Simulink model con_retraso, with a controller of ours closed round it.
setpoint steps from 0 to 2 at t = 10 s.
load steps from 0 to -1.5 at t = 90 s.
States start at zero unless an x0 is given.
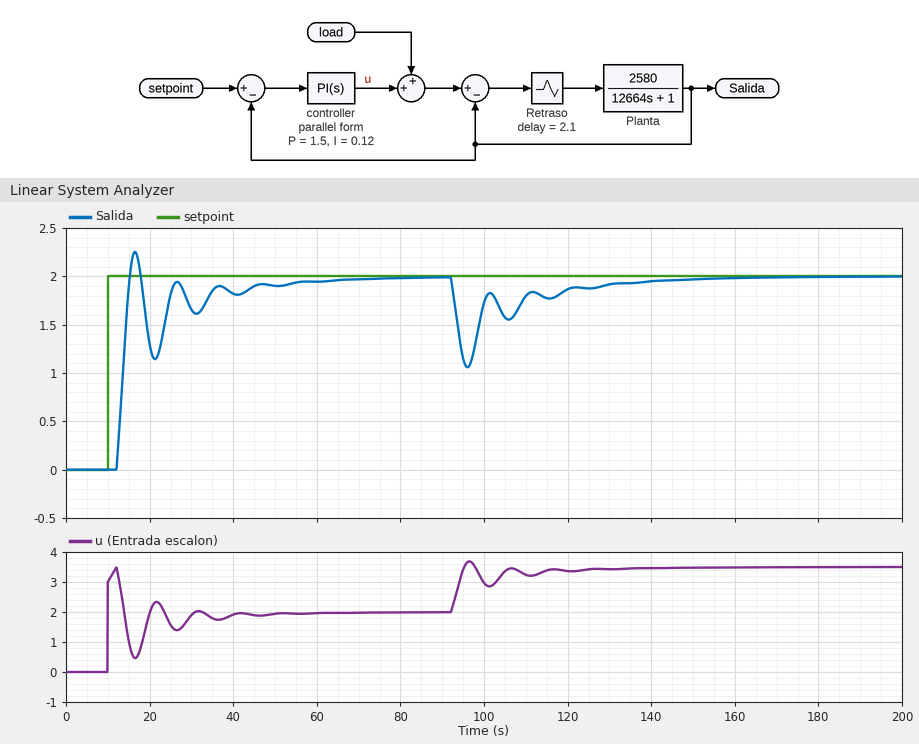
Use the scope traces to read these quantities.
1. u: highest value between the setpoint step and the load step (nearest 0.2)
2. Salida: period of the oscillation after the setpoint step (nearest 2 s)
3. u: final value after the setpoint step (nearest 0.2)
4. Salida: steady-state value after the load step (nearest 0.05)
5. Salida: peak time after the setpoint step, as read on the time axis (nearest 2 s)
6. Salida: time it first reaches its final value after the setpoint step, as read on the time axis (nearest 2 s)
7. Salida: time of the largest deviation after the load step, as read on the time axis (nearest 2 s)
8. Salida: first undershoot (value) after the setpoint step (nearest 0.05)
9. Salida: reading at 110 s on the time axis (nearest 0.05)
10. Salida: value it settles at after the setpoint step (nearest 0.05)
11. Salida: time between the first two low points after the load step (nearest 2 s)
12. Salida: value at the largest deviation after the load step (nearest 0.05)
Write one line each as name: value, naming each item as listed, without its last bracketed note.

u: highest value between the setpoint step and the load step: 3.4
Salida: period of the oscillation after the setpoint step: 10 s
u: final value after the setpoint step: 2.0
Salida: steady-state value after the load step: 2.00
Salida: peak time after the setpoint step, as read on the time axis: 16 s
Salida: time it first reaches its final value after the setpoint step, as read on the time axis: 16 s
Salida: time of the largest deviation after the load step, as read on the time axis: 96 s
Salida: first undershoot (value) after the setpoint step: 1.15
Salida: reading at 110 s on the time axis: 1.80
Salida: value it settles at after the setpoint step: 2.00
Salida: time between the first two low points after the load step: 10 s
Salida: value at the largest deviation after the load step: 1.05
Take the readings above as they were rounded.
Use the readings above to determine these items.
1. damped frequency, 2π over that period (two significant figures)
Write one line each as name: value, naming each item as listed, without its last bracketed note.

damped frequency, 2π over that period: 0.63 rad/s
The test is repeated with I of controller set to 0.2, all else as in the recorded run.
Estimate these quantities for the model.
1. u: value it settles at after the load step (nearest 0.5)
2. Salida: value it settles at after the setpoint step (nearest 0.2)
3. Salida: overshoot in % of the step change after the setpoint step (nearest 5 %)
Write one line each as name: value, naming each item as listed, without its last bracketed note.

u: value it settles at after the load step: 3.5
Salida: value it settles at after the setpoint step: 2.0
Salida: overshoot in % of the step change after the setpoint step: 25 %
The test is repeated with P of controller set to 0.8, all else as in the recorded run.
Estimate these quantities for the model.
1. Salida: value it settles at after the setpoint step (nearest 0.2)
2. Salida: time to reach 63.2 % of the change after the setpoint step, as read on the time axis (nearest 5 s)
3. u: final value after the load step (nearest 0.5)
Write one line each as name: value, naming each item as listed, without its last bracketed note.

Salida: value it settles at after the setpoint step: 2.0
Salida: time to reach 63.2 % of the change after the setpoint step, as read on the time axis: 15 s
u: final value after the load step: 3.5
